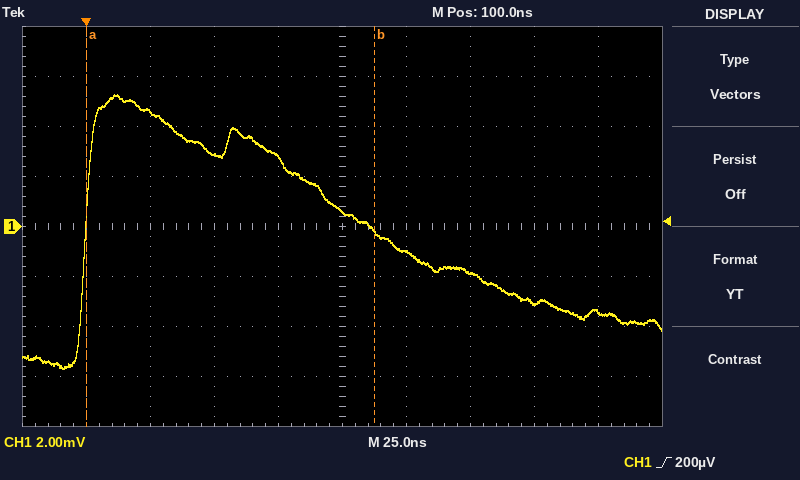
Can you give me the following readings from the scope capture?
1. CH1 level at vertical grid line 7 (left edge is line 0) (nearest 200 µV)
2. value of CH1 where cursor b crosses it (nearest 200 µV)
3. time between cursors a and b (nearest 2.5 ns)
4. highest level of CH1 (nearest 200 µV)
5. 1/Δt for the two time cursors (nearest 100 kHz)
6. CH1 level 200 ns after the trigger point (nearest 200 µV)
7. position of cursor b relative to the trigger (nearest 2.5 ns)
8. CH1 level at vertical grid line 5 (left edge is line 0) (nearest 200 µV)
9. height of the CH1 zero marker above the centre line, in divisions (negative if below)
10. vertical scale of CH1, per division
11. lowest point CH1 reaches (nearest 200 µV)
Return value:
-1.8 mV
-200 µV
112.5 ns
5.2 mV
8.9 MHz
-3.4 mV
+112.5 ns
600 µV
0.0 div
2 mV
-5.6 mV
